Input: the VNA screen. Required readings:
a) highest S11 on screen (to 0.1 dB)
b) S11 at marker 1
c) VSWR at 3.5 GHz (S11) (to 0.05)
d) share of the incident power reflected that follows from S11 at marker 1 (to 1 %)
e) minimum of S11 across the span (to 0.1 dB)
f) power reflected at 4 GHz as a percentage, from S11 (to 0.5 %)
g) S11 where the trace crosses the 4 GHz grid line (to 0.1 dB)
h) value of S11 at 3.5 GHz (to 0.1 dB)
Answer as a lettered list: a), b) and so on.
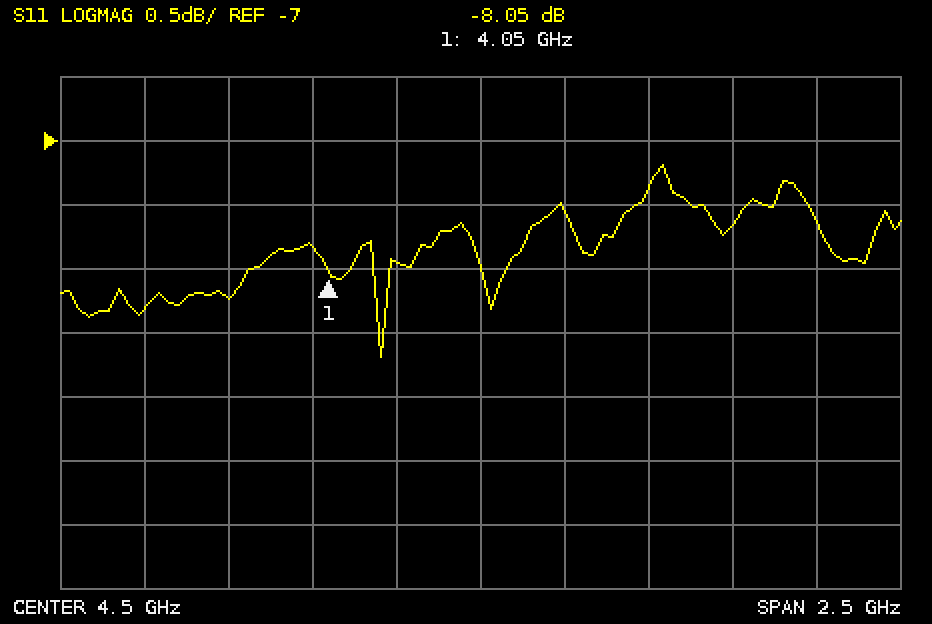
a) -7.2 dB
b) -8.05 dB
c) 2.25
d) 16 %
e) -8.7 dB
f) 16.5 %
g) -7.8 dB
h) -8.3 dB
